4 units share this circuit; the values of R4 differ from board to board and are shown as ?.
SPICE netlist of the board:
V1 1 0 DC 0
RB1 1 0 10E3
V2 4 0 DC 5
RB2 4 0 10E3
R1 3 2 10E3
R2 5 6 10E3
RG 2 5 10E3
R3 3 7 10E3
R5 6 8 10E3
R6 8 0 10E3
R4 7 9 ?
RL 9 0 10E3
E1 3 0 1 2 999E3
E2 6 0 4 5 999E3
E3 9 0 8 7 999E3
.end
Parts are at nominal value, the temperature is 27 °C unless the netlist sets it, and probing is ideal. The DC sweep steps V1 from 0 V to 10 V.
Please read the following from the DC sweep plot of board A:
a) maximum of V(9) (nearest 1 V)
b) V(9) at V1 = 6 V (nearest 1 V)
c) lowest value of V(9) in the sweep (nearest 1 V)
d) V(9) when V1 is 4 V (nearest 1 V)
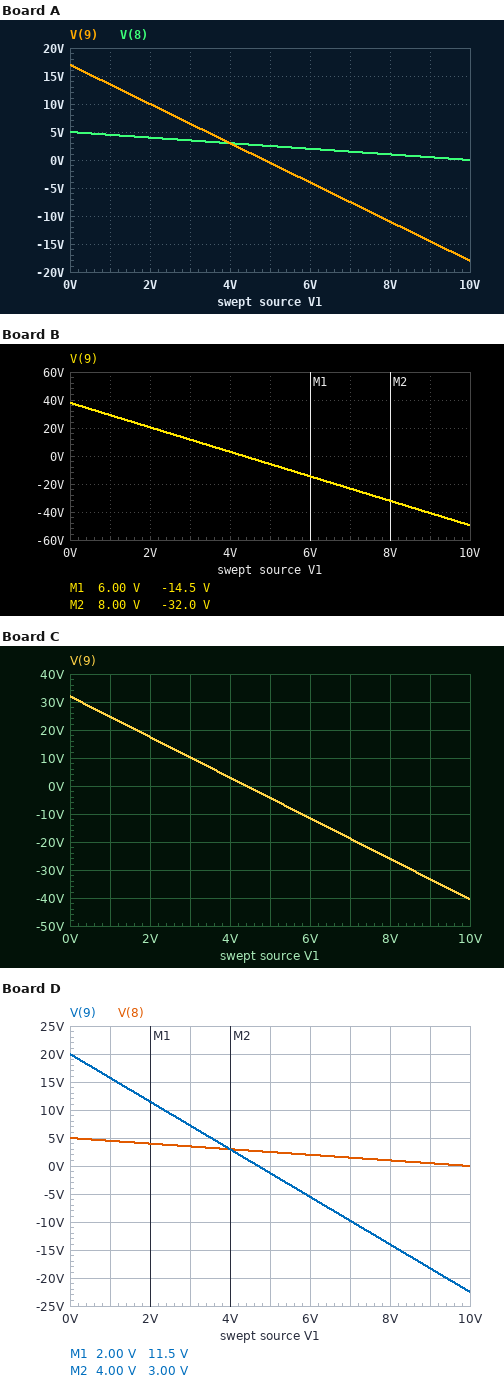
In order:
17 V
-4 V
-18 V
3 V
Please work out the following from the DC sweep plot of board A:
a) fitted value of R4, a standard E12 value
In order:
12 kΩ
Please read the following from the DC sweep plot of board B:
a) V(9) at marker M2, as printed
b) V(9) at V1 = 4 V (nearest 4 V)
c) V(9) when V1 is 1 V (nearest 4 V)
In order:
-32.0 V
4 V
28 V
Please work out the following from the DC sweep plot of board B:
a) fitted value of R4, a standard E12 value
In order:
33 kΩ
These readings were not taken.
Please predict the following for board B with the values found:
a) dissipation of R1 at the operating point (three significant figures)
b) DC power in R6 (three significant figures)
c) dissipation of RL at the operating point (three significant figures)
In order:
2.50 mW
2.50 mW
144 mW
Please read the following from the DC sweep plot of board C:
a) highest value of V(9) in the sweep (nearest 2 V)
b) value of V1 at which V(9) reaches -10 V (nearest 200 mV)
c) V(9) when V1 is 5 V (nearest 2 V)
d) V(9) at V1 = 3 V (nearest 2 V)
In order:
32 V
5.8 V
-4 V
10 V
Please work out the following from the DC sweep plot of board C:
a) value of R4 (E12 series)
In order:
27 kΩ
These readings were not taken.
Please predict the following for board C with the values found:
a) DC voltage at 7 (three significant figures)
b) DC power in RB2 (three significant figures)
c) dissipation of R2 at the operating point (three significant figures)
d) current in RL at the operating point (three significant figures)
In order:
5.00 V
2.50 mW
2.50 mW
3.20 mA
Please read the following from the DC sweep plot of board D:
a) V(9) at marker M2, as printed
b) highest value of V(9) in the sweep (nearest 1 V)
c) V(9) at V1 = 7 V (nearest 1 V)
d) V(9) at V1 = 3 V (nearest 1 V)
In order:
3.00 V
20 V
-10 V
7 V
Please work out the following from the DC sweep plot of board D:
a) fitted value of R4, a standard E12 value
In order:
15 kΩ
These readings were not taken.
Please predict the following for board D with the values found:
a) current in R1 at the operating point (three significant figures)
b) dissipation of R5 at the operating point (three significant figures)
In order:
500 µA
2.50 mW
